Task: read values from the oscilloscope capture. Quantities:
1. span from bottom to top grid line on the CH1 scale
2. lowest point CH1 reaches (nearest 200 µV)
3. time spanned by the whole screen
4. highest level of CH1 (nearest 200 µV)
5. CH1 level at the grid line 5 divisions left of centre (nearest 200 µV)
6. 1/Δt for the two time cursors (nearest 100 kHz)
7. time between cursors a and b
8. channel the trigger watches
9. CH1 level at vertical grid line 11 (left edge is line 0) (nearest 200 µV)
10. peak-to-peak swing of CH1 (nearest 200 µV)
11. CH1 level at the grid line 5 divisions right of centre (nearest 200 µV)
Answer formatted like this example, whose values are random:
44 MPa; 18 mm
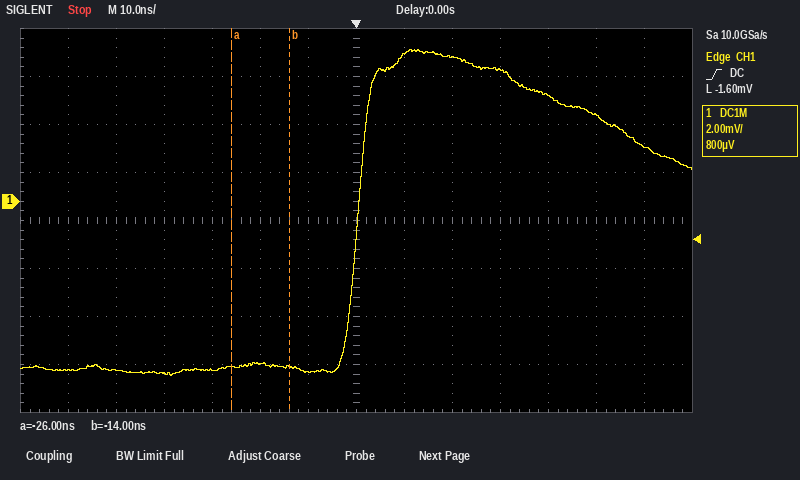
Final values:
16 mV; -7.2 mV; 140 ns; 6.4 mV; -7.0 mV; 83.3 MHz; 12 ns; CH1; 4.4 mV; 13.6 mV; 3.6 mV
